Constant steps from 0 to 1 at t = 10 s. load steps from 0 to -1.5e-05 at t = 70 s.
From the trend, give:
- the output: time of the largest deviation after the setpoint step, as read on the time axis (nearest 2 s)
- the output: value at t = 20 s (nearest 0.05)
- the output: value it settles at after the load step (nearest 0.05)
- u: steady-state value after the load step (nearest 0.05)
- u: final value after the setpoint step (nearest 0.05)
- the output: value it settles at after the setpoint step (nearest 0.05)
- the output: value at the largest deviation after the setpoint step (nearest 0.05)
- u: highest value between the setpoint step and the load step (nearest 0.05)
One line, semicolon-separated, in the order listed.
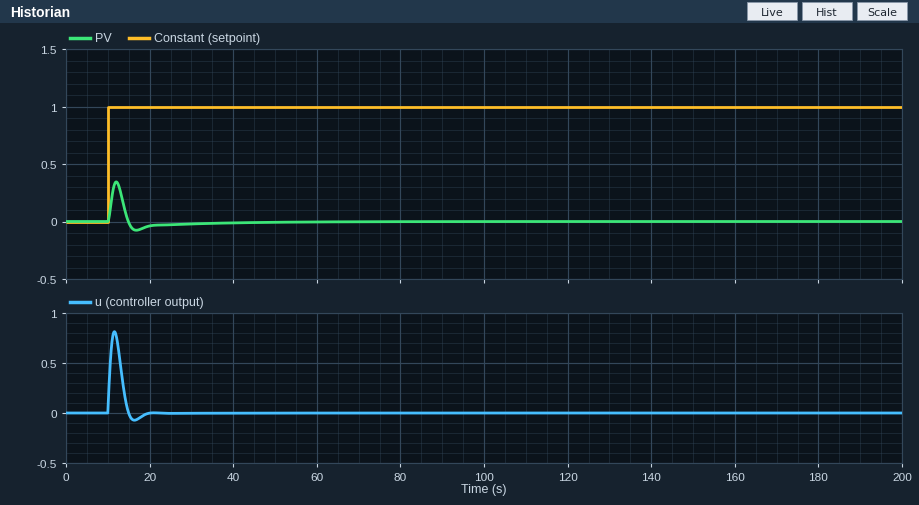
12 s; -0.05; 0.00; 0.00; 0.00; 0.00; 0.35; 0.80
